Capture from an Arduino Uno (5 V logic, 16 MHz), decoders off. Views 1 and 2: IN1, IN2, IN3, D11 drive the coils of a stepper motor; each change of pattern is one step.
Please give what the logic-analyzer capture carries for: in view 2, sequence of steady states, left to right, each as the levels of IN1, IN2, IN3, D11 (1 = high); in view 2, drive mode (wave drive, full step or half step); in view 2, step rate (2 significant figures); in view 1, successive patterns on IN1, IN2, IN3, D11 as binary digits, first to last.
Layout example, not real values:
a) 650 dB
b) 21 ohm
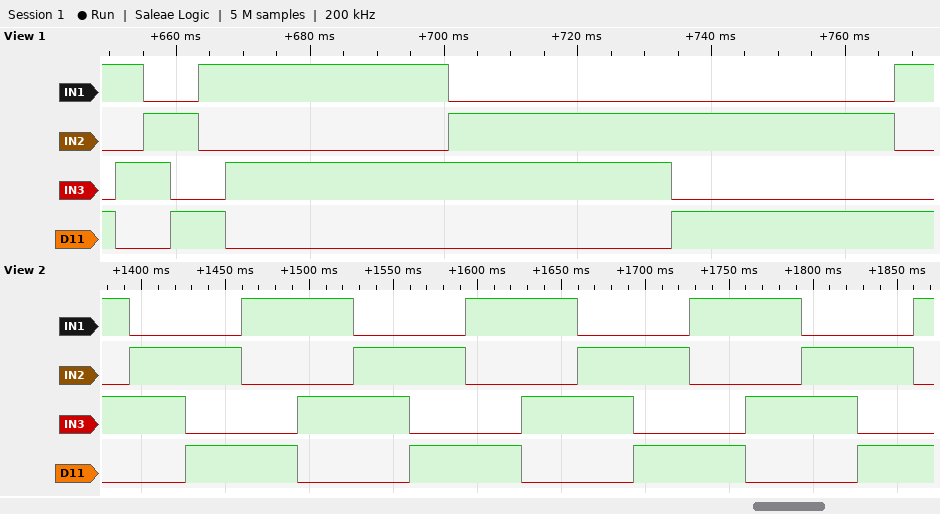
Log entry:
a) 1010 0110 0101 1001 1010 0110 0101 1001 1010 0110 0101 1001 1010 0110 0101 1001
b) full step
c) 30 steps/s
d) 1001 1010 0110 0101 1001 1010 0110 0101 1001
